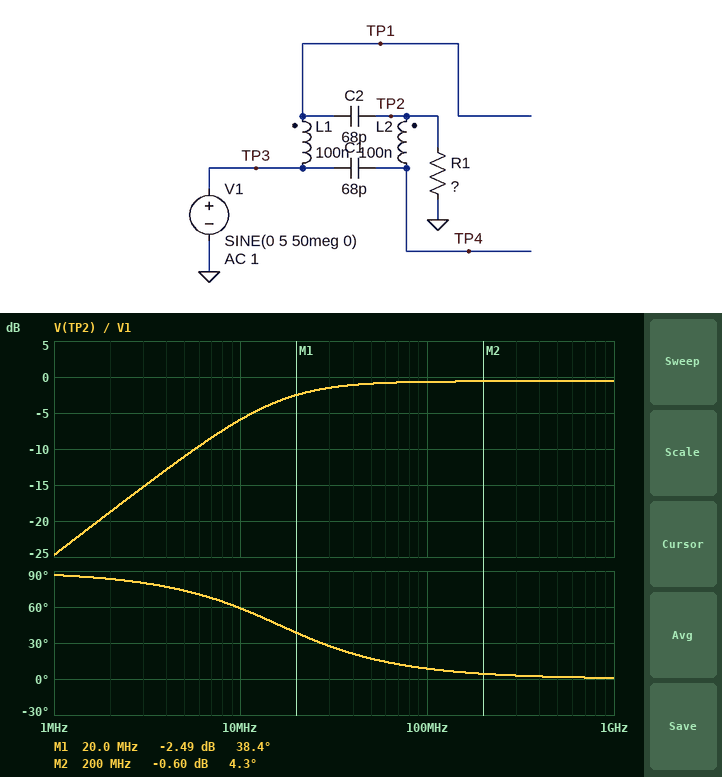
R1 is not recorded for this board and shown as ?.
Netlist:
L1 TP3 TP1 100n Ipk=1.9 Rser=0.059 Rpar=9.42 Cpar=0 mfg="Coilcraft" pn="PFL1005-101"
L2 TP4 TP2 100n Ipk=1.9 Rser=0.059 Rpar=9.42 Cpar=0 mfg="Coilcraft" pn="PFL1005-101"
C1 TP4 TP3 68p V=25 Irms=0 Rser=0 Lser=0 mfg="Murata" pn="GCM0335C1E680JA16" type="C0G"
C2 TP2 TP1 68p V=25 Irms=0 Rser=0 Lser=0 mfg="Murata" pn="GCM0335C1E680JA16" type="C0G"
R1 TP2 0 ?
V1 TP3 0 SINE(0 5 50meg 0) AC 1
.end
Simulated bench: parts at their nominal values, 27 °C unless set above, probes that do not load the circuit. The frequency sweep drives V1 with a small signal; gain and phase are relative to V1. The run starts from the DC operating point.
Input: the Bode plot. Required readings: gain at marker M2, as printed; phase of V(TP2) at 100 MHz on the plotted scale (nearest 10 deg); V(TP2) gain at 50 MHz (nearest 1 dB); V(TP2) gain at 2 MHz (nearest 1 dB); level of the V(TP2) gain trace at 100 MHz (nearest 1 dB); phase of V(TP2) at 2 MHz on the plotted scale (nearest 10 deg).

-0.60 dB
10 deg
-1 dB
-19 dB
-1 dB
80 deg
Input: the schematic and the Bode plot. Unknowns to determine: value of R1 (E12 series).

68 Ω
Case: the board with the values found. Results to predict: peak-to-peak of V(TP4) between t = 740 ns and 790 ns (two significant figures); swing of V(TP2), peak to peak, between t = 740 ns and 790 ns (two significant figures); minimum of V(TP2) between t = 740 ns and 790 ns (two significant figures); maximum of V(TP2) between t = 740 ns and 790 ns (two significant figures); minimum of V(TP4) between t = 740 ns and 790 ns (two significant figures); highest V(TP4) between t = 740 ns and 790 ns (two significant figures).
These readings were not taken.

9.6 V
9.0 V
-4.5 V
4.5 V
-4.8 V
4.8 V
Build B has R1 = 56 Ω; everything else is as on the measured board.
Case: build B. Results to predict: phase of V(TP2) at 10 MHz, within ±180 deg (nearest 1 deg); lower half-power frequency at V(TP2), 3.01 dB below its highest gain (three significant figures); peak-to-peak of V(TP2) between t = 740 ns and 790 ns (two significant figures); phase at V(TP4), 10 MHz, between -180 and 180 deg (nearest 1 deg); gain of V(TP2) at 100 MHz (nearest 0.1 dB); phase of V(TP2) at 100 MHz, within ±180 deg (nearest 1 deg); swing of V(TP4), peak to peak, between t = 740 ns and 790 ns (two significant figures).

63 deg
18.0 MHz
8.7 V
66 deg
-0.8 dB
10 deg
9.4 V
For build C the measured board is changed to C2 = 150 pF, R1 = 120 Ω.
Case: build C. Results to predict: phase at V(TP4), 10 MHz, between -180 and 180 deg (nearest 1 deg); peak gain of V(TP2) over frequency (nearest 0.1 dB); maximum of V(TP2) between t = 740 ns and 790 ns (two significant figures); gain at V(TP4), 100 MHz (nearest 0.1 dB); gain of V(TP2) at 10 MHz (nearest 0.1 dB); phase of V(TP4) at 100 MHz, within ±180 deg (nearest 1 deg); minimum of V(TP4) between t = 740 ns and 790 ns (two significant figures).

31 deg
-0.3 dB
4.8 V
-0.2 dB
-1.4 dB
4 deg
-4.9 V
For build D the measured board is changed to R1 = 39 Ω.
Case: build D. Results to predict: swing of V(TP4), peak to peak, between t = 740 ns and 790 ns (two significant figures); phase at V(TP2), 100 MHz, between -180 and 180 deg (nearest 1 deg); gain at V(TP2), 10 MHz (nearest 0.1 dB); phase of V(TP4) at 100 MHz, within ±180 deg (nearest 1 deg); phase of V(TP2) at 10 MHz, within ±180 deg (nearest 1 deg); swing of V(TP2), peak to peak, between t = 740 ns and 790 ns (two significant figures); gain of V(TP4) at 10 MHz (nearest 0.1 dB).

8.9 V
14 deg
-9.9 dB
15 deg
71 deg
8.0 V
-9.6 dB
